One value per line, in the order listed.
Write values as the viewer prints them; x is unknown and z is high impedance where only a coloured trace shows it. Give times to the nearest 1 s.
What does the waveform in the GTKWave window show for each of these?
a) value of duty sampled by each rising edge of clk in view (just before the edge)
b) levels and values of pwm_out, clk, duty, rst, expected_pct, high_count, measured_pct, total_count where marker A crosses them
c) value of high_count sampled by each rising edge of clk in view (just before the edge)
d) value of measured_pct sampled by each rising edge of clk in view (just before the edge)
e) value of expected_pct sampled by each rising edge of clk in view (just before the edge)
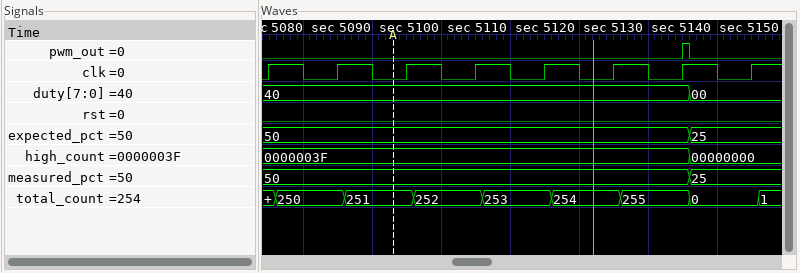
40, 40, 40, 40, 40, 40, 40, 00
pwm_out=0, clk=0, duty=40, rst=0, expected_pct=50, high_count=0000003F, measured_pct=50, total_count=251
0000003F, 0000003F, 0000003F, 0000003F, 0000003F, 0000003F, 0000003F, 00000000
50, 50, 50, 50, 50, 50, 50, 25
50, 50, 50, 50, 50, 50, 50, 25
